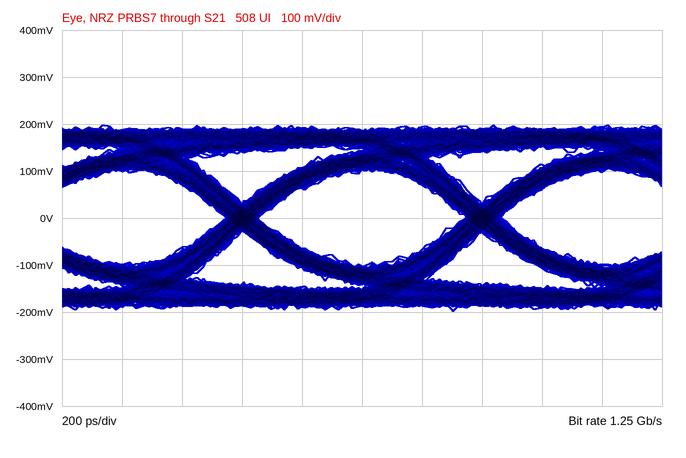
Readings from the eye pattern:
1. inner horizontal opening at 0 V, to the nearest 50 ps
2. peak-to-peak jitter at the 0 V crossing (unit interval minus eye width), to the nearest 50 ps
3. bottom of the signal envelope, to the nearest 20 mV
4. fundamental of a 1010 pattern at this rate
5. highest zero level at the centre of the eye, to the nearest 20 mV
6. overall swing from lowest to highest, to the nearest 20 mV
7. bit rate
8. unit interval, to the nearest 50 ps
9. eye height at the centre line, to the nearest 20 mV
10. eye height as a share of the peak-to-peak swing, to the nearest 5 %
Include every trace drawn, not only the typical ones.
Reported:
700 ps
100 ps
-200 mV
625 MHz
-100 mV
400 mV
1.25 Gb/s
800 ps
200 mV
50 %
